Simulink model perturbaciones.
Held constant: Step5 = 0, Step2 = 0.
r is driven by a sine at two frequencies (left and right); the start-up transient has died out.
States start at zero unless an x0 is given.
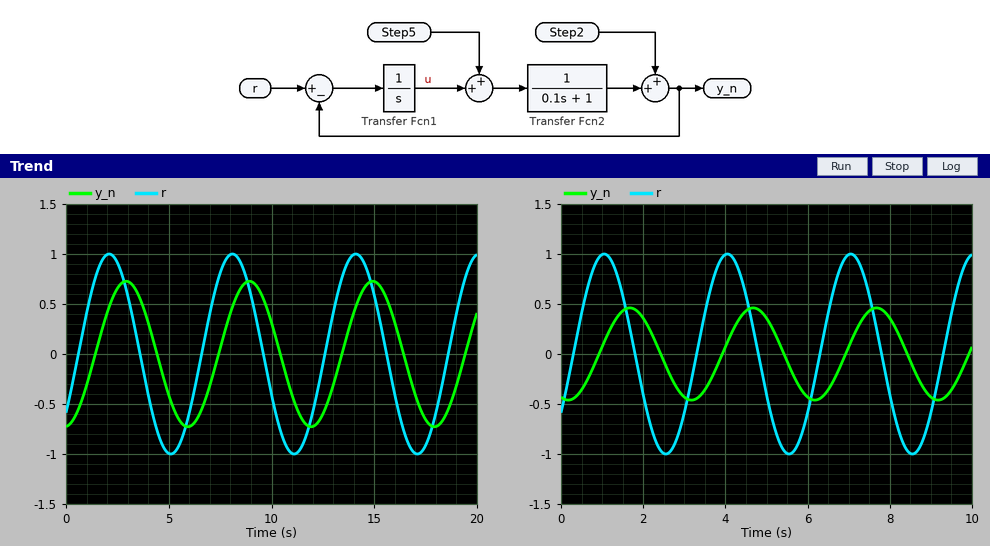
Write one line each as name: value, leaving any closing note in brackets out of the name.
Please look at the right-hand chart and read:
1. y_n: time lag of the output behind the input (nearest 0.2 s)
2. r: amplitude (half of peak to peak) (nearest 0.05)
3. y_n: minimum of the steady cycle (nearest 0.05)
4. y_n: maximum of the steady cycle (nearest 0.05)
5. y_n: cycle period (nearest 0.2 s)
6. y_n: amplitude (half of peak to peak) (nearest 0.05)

y_n: time lag of the output behind the input: 0.6 s
r: amplitude (half of peak to peak): 1.00
y_n: minimum of the steady cycle: -0.45
y_n: maximum of the steady cycle: 0.45
y_n: cycle period: 3.0 s
y_n: amplitude (half of peak to peak): 0.45
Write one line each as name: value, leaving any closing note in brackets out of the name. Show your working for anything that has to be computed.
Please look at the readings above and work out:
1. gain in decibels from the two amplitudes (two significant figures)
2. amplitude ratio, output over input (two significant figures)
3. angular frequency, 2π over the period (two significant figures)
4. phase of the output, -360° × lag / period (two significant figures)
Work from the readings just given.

gain in decibels from the two amplitudes: 20 log10(0.45 / 1) = -6.9 dB
amplitude ratio, output over input: 0.45 / 1 = 0.45
angular frequency, 2π over the period: 2π / 3 = 2.1 rad/s
phase of the output, -360° × lag / period: -360 × 0.6 / 3 = -72°
